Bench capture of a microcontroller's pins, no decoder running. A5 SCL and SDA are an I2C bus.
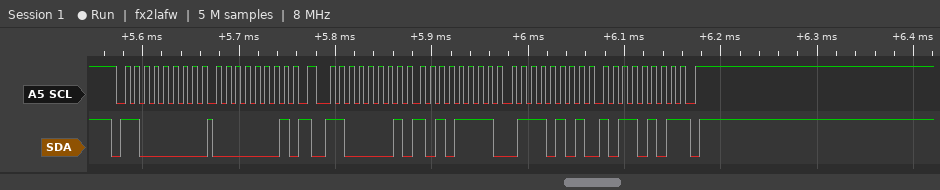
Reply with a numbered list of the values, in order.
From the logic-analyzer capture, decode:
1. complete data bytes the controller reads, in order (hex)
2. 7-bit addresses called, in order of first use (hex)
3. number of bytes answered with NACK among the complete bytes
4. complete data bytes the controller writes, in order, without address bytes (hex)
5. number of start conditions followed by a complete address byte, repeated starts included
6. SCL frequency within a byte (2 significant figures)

1. AF 75 B5
2. 0x60
3. 1
4. 01
5. 2
6. 100 kHz
